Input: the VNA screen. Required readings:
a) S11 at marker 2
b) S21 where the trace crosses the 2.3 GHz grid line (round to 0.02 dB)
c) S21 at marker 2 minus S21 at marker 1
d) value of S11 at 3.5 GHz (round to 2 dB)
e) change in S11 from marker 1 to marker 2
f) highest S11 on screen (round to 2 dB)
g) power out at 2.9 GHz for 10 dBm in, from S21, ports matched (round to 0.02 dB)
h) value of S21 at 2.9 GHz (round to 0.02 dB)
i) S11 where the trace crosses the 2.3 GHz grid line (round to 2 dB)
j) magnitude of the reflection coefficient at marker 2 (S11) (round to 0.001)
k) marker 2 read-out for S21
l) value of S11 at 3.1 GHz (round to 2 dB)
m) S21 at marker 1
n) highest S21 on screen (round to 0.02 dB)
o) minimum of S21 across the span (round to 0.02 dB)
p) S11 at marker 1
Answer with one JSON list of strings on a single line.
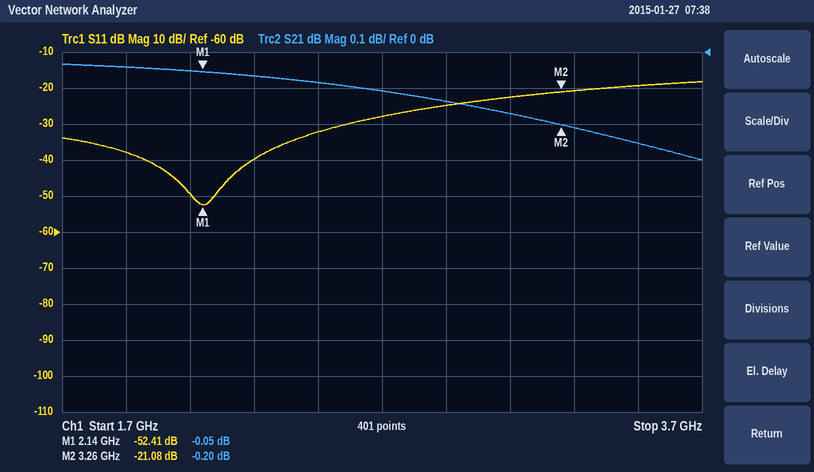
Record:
["-21.08 dB", "-0.06 dB", "-0.15 dB", "-20 dB", "31.33 dB", "-18 dB", "9.86 dBm", "-0.14 dB", "-40 dB", "0.088", "-0.20 dB", "-22 dB", "-0.05 dB", "-0.04 dB", "-0.30 dB", "-52.41 dB"]
